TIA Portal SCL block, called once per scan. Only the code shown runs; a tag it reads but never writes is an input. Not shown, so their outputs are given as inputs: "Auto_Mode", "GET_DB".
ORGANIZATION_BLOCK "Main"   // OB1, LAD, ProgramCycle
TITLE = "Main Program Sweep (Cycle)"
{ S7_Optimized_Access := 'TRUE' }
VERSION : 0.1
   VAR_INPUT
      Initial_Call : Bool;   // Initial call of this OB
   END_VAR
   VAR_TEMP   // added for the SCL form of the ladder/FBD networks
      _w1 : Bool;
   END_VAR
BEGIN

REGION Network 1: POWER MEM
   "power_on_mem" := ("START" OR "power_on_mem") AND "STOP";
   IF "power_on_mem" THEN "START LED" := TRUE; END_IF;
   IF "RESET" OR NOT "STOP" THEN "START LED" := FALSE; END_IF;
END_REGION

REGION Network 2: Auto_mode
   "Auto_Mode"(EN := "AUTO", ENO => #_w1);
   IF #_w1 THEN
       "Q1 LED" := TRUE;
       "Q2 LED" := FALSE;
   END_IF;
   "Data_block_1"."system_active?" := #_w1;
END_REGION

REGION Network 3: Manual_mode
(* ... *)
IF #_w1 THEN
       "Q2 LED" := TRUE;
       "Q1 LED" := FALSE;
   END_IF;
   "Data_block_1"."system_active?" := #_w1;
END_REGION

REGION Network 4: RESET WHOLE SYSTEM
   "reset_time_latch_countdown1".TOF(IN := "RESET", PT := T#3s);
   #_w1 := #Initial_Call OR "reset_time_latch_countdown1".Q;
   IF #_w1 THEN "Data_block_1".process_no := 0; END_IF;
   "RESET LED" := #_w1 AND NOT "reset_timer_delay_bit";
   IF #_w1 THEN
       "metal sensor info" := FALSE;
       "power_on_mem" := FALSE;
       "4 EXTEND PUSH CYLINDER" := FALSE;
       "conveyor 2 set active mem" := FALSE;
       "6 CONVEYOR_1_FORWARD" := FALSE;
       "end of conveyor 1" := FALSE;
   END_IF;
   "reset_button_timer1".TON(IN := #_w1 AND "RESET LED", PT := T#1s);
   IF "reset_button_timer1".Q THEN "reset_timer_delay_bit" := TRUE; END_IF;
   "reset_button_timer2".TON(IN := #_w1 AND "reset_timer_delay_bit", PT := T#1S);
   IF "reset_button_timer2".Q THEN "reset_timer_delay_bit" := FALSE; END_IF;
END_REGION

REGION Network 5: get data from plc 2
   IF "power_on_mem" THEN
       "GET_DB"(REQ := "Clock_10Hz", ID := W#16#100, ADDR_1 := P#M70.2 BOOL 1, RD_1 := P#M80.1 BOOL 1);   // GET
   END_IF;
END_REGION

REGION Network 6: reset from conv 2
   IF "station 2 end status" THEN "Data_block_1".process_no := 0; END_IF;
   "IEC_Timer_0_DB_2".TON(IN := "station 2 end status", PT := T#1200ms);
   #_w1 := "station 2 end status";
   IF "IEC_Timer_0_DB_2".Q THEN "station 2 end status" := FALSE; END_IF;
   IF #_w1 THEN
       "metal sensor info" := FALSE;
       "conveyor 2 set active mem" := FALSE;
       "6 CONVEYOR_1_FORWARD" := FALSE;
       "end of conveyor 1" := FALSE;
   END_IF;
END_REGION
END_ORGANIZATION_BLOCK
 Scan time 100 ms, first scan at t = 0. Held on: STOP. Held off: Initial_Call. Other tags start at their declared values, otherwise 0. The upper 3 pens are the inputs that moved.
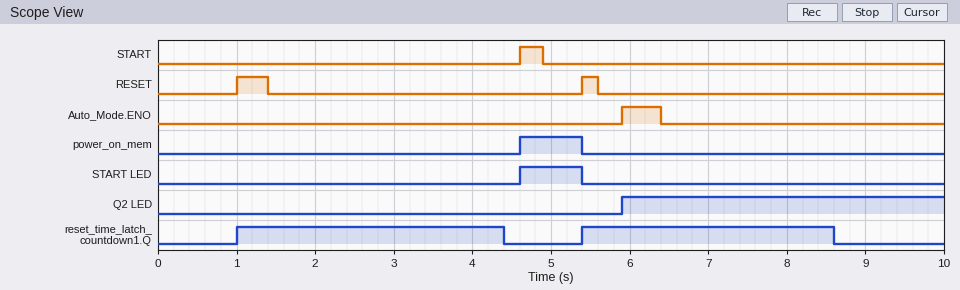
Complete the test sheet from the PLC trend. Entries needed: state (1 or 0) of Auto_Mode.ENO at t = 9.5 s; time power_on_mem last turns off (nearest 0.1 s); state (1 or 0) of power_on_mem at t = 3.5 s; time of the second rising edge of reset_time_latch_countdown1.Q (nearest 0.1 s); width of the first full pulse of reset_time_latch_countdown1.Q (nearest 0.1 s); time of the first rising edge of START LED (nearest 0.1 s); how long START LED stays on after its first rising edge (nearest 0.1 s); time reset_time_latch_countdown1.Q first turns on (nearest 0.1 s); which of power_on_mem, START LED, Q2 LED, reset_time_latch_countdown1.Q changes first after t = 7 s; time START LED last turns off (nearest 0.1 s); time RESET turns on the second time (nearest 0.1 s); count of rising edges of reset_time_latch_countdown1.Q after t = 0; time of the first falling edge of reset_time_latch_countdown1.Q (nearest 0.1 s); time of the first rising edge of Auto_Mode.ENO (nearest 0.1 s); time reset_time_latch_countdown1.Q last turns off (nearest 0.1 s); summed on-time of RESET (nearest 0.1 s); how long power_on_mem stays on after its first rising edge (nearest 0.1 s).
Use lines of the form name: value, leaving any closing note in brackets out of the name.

state (1 or 0) of Auto_Mode.ENO at t = 9.5 s: 0
time power_on_mem last turns off: 5.4 s
state (1 or 0) of power_on_mem at t = 3.5 s: 0
time of the second rising edge of reset_time_latch_countdown1.Q: 5.4 s
width of the first full pulse of reset_time_latch_countdown1.Q: 3.4 s
time of the first rising edge of START LED: 4.6 s
how long START LED stays on after its first rising edge: 0.8 s
time reset_time_latch_countdown1.Q first turns on: 1.0 s
which of power_on_mem, START LED, Q2 LED, reset_time_latch_countdown1.Q changes first after t = 7 s: reset_time_latch_countdown1.Q
time START LED last turns off: 5.4 s
time RESET turns on the second time: 5.4 s
count of rising edges of reset_time_latch_countdown1.Q after t = 0: 2
time of the first falling edge of reset_time_latch_countdown1.Q: 4.4 s
time of the first rising edge of Auto_Mode.ENO: 5.9 s
time reset_time_latch_countdown1.Q last turns off: 8.6 s
summed on-time of RESET: 0.6 s
how long power_on_mem stays on after its first rising edge: 0.8 s
